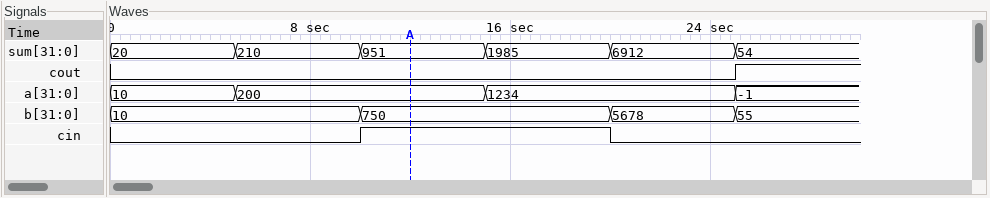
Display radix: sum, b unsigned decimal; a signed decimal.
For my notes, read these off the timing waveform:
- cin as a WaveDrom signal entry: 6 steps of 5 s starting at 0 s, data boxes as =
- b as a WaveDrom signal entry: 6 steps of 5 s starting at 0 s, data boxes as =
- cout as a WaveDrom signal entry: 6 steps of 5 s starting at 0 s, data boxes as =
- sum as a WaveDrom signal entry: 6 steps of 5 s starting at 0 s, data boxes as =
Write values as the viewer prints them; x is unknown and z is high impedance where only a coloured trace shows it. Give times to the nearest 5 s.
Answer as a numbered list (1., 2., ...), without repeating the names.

1. {name: 'cin', wave: '0.1.0.'}
2. {name: 'b', wave: '=.=.==', data: '10 750 5678 55'}
3. {name: 'cout', wave: '0....1'}
4. {name: 'sum', wave: '======', data: '20 210 951 1985 6912 54'}
